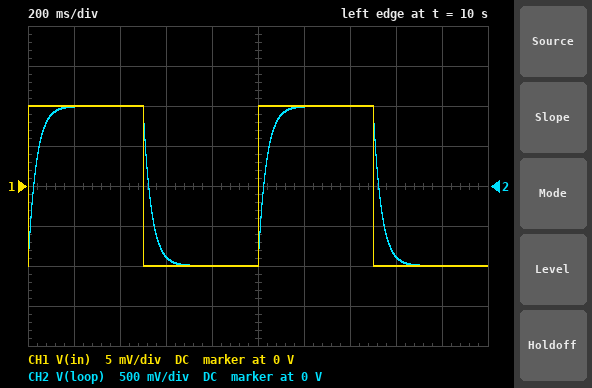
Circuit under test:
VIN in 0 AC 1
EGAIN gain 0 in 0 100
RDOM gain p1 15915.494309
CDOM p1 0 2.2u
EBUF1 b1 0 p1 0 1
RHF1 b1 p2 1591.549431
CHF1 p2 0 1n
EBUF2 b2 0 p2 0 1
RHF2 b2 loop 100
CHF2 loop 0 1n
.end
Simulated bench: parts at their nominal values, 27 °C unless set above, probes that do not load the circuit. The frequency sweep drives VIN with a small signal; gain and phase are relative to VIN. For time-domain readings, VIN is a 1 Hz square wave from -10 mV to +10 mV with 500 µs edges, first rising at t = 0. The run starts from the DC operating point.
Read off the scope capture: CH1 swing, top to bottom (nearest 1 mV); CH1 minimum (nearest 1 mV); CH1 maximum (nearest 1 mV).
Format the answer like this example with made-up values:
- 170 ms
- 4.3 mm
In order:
- 20 mV
- -10 mV
- 10 mV
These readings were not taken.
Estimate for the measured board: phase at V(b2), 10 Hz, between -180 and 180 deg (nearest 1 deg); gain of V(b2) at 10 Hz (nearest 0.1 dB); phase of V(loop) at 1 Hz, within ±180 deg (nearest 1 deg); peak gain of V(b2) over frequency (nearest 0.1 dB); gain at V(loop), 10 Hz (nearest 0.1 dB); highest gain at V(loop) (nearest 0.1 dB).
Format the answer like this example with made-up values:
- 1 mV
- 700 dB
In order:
- -66 deg
- 32.3 dB
- -12 deg
- 40.0 dB
- 32.3 dB
- 40.0 dB
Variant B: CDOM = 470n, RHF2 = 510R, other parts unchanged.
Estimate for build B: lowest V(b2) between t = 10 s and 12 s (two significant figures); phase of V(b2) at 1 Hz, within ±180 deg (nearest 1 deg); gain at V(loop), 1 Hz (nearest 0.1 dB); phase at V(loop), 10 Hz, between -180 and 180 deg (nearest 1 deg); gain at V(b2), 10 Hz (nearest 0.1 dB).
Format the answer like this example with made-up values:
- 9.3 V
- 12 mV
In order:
- -1.0 V
- -3 deg
- 40.0 dB
- -25 deg
- 39.1 dB
